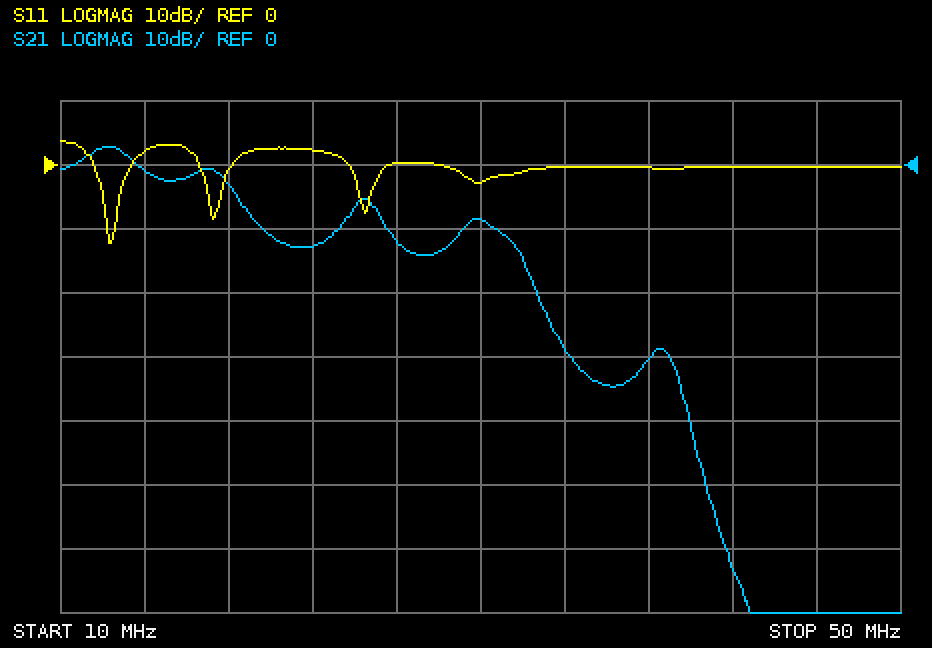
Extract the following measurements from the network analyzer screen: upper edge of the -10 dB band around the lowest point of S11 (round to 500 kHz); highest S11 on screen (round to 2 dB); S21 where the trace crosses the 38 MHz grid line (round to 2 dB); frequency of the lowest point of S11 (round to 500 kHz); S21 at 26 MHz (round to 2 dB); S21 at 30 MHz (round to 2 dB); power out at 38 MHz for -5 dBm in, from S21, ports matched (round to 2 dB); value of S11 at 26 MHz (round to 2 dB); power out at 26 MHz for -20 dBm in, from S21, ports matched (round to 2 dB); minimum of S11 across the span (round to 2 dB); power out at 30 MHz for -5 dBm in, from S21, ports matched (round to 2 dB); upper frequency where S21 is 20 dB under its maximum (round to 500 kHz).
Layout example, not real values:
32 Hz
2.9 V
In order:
12.5 MHz
4 dB
-30 dB
12.5 MHz
-12 dB
-8 dB
-36 dBm
0 dB
-32 dBm
-12 dB
-14 dBm
32.5 MHz
